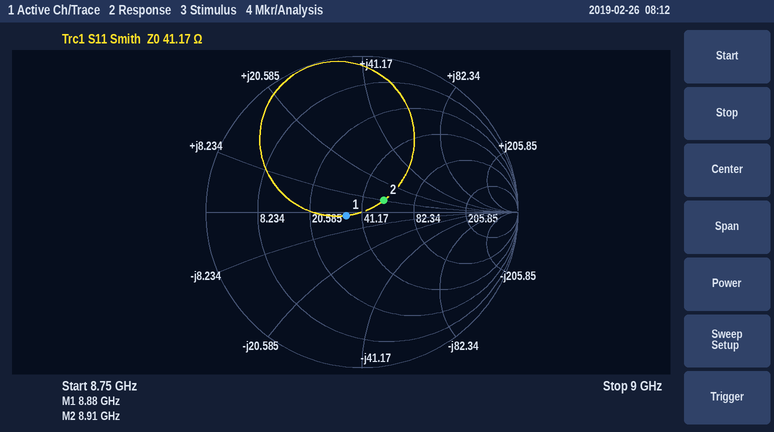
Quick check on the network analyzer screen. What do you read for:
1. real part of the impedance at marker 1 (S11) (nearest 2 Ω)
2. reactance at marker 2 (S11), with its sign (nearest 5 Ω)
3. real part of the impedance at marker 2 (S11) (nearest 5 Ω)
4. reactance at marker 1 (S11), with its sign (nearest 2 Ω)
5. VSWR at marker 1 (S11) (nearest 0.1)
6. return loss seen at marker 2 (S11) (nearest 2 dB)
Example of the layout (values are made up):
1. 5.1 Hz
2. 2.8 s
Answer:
1. 34 Ω
2. +10 Ω
3. 55 Ω
4. -2 Ω
5. 1.2
6. 16 dB
